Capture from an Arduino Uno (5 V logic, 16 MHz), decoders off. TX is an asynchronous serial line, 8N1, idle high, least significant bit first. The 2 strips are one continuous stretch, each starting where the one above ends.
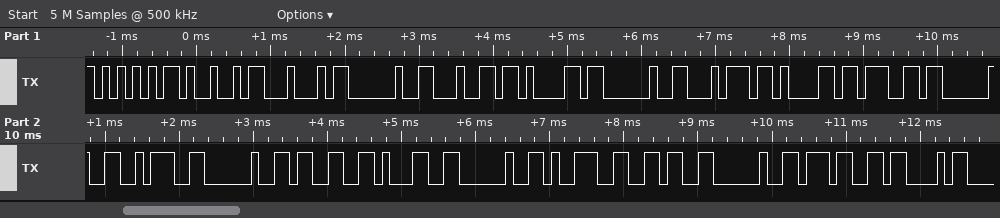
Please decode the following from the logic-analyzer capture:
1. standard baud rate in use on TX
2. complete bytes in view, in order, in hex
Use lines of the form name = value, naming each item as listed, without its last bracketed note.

standard baud rate in use on TX = 9600 baud
complete bytes in view, in order, in hex = 0x55 0x49 0x44 0x20 0x64 0x61 0x20 0x74 0x61 0x67 0x20 0x3A 0x20 0x33 0x31 0x20 0x39 0x36 0x20 0x37 0x43
